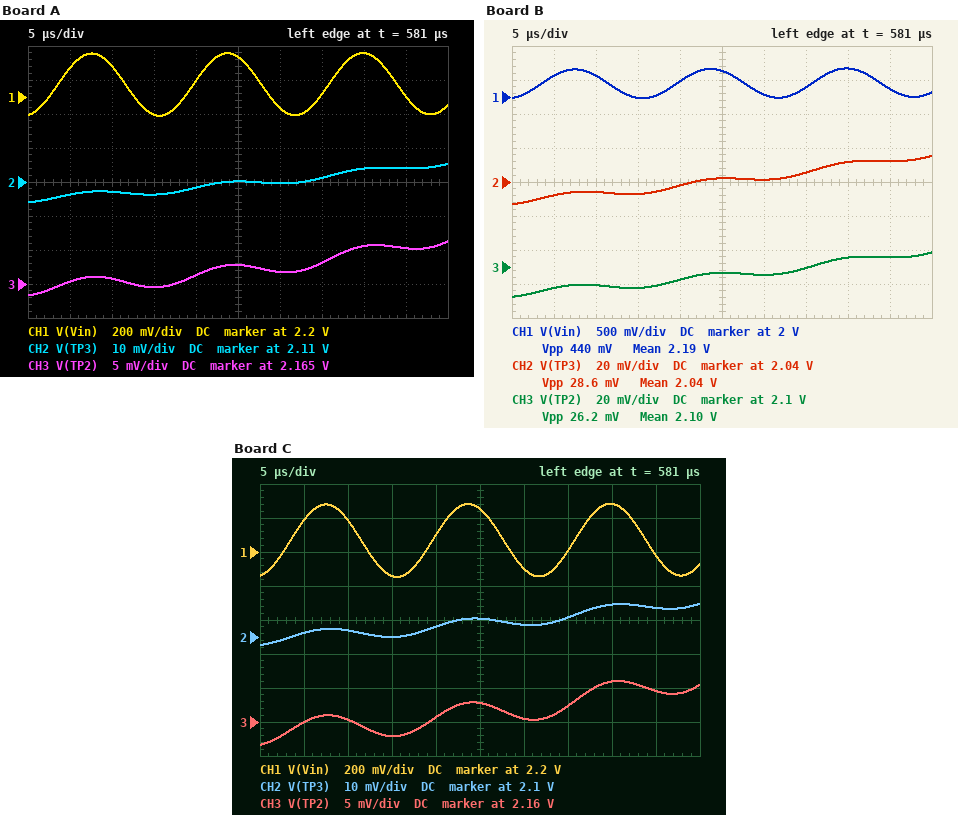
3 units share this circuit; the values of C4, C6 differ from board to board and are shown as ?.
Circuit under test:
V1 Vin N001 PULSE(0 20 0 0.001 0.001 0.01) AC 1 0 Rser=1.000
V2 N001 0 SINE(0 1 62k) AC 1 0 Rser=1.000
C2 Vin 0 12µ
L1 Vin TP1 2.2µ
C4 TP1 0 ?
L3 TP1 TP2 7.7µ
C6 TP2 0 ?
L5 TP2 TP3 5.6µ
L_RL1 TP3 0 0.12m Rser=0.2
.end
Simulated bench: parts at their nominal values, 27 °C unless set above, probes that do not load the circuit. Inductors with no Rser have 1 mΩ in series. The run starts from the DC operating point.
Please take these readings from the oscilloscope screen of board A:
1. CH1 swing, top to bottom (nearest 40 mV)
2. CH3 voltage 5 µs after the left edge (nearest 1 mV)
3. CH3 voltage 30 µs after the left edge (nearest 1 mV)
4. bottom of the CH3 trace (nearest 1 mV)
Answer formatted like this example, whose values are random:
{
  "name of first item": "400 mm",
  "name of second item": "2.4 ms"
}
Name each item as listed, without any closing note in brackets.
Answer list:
{
  "CH1 swing, top to bottom": "360 mV",
  "CH3 voltage 5 µs after the left edge": "2.165 V",
  "CH3 voltage 30 µs after the left edge": "2.167 V",
  "bottom of the CH3 trace": "2.163 V"
}
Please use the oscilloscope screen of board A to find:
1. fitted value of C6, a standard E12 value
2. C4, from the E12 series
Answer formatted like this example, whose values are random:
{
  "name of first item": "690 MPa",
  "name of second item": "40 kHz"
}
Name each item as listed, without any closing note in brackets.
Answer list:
{
  "fitted value of C6, a standard E12 value": "100 µF",
  "C4, from the E12 series": "8.2 µF"
}
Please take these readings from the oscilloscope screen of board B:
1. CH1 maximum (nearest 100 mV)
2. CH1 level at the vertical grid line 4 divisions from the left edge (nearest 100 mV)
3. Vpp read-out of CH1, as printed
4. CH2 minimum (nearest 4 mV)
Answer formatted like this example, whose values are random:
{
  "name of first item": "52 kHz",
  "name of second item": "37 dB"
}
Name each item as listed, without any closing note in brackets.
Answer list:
{
  "CH1 maximum": "2.4 V",
  "CH1 level at the vertical grid line 4 divisions from the left edge": "2.2 V",
  "Vpp read-out of CH1, as printed": "440 mV",
  "CH2 minimum": "2.028 V"
}
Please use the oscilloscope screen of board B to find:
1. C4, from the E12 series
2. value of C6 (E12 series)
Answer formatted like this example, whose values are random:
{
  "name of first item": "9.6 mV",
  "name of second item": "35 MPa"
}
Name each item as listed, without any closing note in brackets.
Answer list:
{
  "C4, from the E12 series": "6.8 µF",
  "value of C6": "82 µF"
}
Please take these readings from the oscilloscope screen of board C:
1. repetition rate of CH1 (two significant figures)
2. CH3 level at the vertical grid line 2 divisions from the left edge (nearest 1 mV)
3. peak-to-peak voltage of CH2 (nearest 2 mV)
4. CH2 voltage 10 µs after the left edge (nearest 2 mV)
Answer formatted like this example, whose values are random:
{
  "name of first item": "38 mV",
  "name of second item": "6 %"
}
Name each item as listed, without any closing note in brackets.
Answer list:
{
  "repetition rate of CH1": "62 kHz",
  "CH3 level at the vertical grid line 2 divisions from the left edge": "2.160 V",
  "peak-to-peak voltage of CH2": "12 mV",
  "CH2 voltage 10 µs after the left edge": "2.102 V"
}
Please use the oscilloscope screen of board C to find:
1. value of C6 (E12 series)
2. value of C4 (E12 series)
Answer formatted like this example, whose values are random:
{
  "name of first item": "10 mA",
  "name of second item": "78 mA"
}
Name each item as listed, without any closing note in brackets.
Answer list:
{
  "value of C6": "100 µF",
  "value of C4": "6.8 µF"
}
